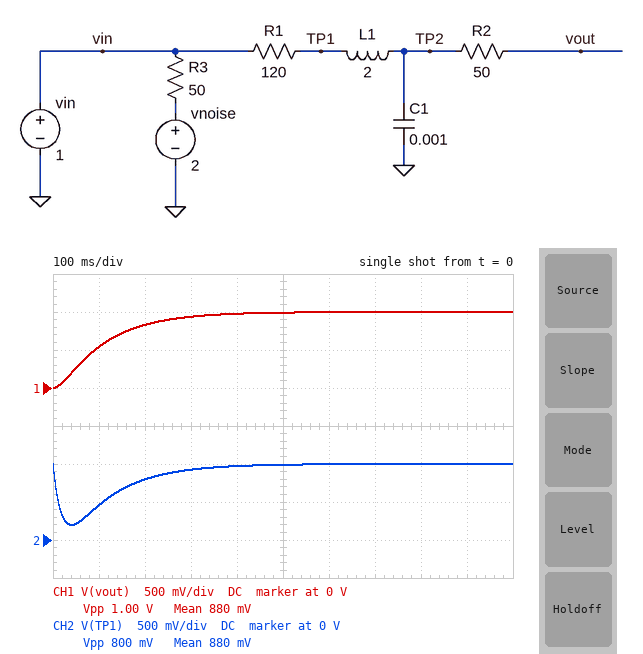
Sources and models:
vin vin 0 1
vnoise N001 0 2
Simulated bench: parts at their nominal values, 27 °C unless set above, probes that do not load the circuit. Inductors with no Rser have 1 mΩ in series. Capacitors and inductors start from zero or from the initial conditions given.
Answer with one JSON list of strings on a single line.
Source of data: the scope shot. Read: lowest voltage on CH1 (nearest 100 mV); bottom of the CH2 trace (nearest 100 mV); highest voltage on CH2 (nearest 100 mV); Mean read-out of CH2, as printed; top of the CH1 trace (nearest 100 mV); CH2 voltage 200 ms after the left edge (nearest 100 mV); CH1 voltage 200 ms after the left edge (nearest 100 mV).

["0 V", "200 mV", "1.0 V", "880 mV", "1.0 V", "800 mV", "800 mV"]
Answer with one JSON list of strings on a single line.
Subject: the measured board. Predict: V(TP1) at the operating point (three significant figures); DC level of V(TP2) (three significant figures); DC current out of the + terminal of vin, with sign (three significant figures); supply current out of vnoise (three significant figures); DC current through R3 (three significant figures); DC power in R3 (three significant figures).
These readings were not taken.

["1.00 V", "1.00 V", "-20.0 mA", "20.0 mA", "20.0 mA", "20.0 mW"]
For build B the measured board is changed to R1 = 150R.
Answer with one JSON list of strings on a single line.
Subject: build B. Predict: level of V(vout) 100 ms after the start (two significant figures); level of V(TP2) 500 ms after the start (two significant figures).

["460 mV", "970 mV"]
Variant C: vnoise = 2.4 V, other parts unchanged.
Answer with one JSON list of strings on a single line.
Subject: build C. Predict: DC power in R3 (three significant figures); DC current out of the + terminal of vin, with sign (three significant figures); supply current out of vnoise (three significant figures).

["39.2 mW", "-28.0 mA", "28.0 mA"]
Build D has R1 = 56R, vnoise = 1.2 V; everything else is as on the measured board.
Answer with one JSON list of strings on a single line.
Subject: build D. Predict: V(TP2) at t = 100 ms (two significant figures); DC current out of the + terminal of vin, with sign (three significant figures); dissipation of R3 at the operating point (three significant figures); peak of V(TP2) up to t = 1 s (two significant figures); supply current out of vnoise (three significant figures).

["850 mV", "-4.00 mA", "800 µW", "1.1 V", "4.00 mA"]
